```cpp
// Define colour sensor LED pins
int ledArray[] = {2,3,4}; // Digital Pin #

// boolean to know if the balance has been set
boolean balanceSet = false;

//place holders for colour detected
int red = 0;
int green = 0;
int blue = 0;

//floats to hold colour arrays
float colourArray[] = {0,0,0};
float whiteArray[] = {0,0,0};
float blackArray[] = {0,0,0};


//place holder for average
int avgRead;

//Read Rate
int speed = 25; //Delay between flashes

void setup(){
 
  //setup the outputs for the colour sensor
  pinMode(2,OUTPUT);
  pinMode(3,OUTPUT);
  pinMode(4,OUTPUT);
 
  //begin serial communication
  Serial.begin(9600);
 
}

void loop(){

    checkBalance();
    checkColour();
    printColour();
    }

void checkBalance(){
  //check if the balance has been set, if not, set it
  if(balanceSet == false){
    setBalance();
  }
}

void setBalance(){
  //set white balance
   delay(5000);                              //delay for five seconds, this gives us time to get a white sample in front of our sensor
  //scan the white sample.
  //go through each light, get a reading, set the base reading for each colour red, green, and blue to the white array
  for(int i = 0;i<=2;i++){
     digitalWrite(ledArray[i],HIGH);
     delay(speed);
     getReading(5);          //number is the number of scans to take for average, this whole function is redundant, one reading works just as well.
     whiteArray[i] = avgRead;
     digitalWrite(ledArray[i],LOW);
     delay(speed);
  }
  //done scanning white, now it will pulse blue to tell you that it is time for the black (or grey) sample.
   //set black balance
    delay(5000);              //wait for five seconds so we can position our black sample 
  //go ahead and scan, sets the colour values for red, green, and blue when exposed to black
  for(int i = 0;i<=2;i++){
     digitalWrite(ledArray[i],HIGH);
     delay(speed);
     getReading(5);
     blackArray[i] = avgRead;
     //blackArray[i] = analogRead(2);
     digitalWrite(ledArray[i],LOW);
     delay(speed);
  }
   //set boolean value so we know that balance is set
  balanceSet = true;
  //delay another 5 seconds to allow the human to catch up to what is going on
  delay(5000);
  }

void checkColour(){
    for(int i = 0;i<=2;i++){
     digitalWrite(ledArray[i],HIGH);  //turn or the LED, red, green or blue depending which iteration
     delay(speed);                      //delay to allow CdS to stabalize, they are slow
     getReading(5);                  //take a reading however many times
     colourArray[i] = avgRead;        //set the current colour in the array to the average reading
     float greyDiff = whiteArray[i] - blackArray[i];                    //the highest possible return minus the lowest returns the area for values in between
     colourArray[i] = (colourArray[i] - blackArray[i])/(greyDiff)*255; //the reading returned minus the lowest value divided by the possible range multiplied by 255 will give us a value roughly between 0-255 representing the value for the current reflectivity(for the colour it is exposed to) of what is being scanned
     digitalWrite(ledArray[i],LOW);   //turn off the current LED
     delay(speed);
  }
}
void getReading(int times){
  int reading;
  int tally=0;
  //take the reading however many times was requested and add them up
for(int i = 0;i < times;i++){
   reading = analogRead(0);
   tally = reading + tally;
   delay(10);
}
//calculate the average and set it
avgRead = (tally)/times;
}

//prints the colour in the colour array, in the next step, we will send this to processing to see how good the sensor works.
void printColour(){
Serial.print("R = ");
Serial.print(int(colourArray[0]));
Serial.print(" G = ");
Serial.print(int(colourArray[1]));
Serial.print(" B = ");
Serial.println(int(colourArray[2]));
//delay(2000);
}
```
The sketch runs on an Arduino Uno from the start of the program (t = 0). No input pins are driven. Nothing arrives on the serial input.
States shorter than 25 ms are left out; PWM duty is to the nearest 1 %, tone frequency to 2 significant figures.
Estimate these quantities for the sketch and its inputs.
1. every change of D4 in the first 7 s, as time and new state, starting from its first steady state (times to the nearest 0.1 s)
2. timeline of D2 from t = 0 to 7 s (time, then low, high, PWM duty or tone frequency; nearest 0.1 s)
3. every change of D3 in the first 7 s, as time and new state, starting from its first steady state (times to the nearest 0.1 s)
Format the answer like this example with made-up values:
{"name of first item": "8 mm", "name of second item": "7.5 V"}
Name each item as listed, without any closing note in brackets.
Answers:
{"every change of D4 in the first 7 s, as time and new state, starting from its first steady state": "0 s low; 5.2 s high; 5.3 s low", "timeline of D2 from t = 0 to 7 s": "0 s low; 5 s high; 5.1 s low", "every change of D3 in the first 7 s, as time and new state, starting from its first steady state": "0 s low; 5.1 s high; 5.2 s low"}
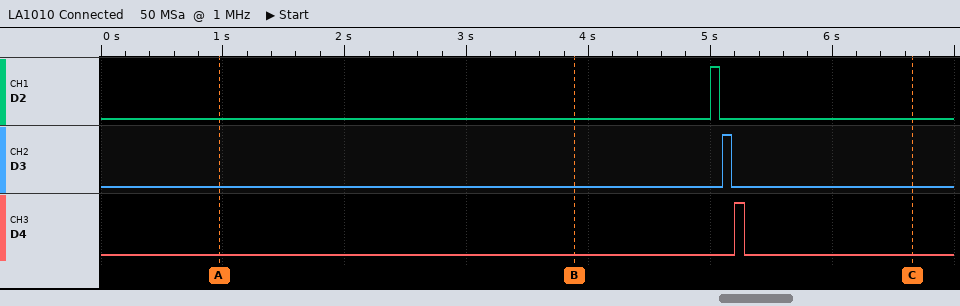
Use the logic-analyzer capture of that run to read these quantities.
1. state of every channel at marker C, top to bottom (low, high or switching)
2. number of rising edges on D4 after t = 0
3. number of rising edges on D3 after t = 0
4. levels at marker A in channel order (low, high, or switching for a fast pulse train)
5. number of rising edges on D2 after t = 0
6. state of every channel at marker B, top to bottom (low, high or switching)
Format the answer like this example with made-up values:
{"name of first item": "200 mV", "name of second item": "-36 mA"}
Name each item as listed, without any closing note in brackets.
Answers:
{"state of every channel at marker C, top to bottom": "D2 low, D3 low, D4 low", "number of rising edges on D4 after t = 0": "1", "number of rising edges on D3 after t = 0": "1", "levels at marker A in channel order": "D2 low, D3 low, D4 low", "number of rising edges on D2 after t = 0": "1", "state of every channel at marker B, top to bottom": "D2 low, D3 low, D4 low"}
